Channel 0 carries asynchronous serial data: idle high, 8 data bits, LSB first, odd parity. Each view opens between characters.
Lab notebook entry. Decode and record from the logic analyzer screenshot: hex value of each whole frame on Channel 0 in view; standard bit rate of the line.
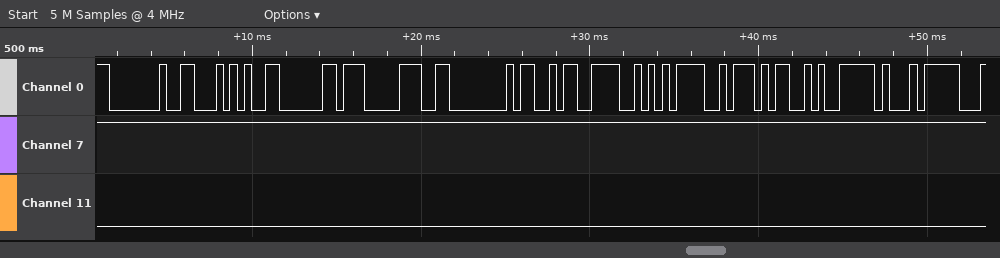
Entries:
40, 54, 60, 70, 80, 9A, AA, BA, CA, D1
2400 baud
